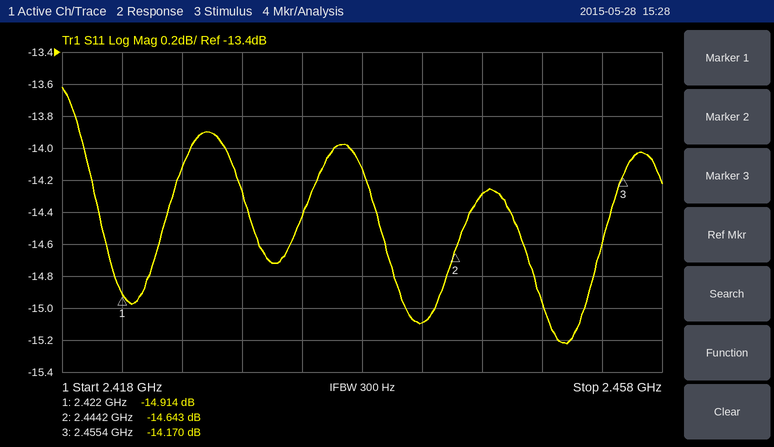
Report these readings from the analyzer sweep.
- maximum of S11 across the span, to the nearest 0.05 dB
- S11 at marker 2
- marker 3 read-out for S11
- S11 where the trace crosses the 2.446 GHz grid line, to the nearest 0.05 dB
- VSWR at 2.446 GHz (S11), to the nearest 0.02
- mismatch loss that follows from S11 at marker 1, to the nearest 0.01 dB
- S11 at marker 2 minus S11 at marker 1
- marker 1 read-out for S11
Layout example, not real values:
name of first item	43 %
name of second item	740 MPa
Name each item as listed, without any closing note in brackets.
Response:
maximum of S11 across the span, to the nearest 0.05 dB	-13.60 dB
S11 at marker 2	-14.643 dB
marker 3 read-out for S11	-14.170 dB
S11 where the trace crosses the 2.446 GHz grid line, to the nearest 0.05 dB	-14.30 dB
VSWR at 2.446 GHz (S11), to the nearest 0.02	1.48
mismatch loss that follows from S11 at marker 1, to the nearest 0.01 dB	0.14 dB
S11 at marker 2 minus S11 at marker 1	0.271 dB
marker 1 read-out for S11	-14.914 dB
